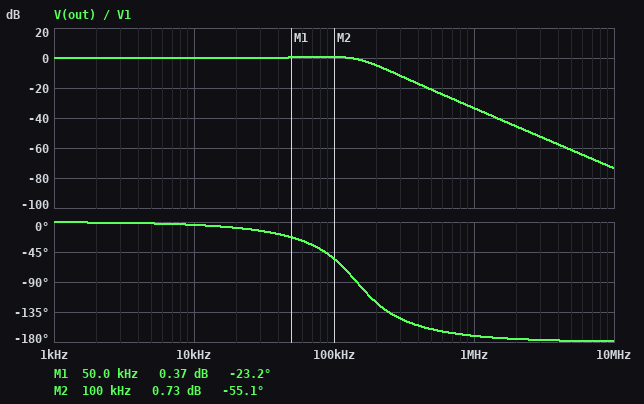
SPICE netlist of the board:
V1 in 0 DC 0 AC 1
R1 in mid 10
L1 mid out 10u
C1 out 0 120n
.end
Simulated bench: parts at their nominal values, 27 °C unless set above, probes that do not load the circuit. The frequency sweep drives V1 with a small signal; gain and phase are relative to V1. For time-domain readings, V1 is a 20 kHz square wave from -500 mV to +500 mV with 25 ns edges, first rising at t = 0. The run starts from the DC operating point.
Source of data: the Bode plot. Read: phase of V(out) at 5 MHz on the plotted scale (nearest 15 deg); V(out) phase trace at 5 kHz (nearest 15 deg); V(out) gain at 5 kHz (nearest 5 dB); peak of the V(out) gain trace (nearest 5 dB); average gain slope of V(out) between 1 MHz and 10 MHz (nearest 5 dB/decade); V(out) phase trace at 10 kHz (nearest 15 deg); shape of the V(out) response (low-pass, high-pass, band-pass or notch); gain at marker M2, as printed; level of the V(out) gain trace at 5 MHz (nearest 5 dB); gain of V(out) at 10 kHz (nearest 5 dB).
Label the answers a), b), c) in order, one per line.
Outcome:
a) -180 deg
b) 0 deg
c) 0 dB
d) 0 dB
e) -40 dB/decade
f) 0 deg
g) low-pass
h) 0.73 dB
i) -60 dB
j) 0 dB
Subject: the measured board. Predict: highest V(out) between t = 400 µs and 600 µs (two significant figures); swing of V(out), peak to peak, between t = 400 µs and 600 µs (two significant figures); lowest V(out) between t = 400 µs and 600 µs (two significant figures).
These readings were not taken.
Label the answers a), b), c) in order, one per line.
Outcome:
a) 630 mV
b) 1.3 V
c) -630 mV
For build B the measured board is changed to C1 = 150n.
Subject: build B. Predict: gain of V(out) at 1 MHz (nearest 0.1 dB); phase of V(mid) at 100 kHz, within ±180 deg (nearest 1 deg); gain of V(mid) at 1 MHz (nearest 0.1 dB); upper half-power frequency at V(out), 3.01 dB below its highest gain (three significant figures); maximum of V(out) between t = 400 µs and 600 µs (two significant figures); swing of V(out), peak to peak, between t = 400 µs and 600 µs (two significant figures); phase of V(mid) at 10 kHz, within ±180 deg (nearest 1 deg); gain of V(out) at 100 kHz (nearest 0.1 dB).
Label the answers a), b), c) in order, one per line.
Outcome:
a) -35.4 dB
b) -67 deg
c) -0.1 dB
d) 143 kHz
e) 590 mV
f) 1.2 V
g) -5 deg
h) -0.2 dB
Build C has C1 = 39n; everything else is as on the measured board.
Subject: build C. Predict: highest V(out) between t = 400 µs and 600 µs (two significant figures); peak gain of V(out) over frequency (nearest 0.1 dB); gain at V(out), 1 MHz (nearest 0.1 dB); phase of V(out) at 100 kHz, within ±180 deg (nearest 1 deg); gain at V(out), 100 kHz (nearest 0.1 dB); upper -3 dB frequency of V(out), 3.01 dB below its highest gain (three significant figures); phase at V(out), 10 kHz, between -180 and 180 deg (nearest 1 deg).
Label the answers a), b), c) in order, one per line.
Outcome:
a) 860 mV
b) 4.5 dB
c) -23.3 dB
d) -16 deg
e) 1.1 dB
f) 301 kHz
g) -1 deg
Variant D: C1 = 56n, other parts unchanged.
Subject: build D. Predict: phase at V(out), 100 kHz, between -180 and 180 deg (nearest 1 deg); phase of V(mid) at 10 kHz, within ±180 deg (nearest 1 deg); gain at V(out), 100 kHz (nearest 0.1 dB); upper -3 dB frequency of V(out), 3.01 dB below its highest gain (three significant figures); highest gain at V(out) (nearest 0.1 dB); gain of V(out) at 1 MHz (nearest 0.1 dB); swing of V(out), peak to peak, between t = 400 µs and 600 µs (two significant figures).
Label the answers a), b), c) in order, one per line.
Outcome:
a) -24 deg
b) -2 deg
c) 1.4 dB
d) 253 kHz
e) 3.2 dB
f) -26.6 dB
g) 1.6 V
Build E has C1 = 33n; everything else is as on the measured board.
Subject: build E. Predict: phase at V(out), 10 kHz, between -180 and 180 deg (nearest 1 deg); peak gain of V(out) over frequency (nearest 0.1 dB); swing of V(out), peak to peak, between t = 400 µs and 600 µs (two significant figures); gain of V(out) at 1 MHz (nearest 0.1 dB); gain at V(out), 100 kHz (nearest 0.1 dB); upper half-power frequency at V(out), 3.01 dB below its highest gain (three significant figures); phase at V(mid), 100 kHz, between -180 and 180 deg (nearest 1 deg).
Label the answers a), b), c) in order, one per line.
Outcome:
a) -1 deg
b) 5.2 dB
c) 1.8 V
d) -21.7 dB
e) 1.0 dB
f) 326 kHz
g) -13 deg
